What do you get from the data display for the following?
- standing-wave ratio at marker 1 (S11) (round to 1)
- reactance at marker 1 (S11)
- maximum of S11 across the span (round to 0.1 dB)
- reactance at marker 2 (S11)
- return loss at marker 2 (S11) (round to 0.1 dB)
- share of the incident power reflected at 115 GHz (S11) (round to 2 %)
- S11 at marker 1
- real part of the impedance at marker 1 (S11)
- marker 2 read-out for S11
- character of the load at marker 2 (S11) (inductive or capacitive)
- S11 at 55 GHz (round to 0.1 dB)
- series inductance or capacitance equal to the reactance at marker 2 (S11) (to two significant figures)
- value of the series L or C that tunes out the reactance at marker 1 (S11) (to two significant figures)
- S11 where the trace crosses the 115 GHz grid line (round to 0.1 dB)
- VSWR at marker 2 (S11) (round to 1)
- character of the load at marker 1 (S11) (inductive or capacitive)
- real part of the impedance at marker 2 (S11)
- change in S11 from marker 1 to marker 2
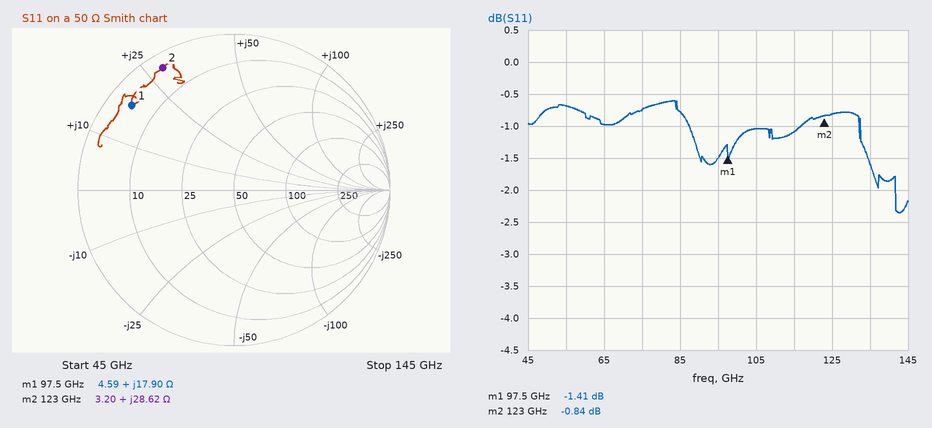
12
+17.90 Ω
-0.6 dB
+28.62 Ω
0.8 dB
78 %
-1.41 dB
4.59 Ω
-0.84 dB
inductive
-0.7 dB
37 pH
91 fF
-1.1 dB
21
inductive
3.20 Ω
0.57 dB
